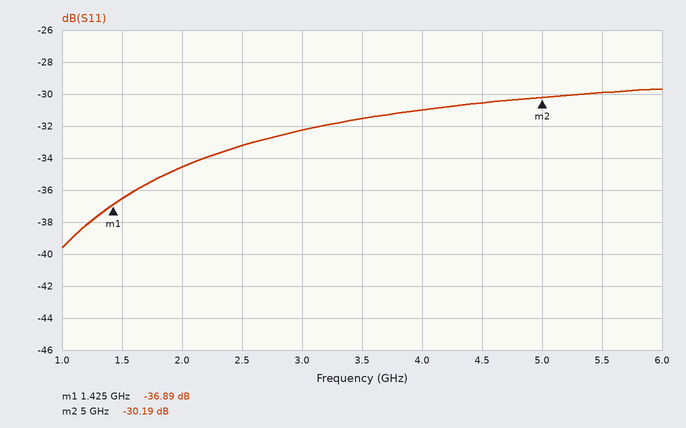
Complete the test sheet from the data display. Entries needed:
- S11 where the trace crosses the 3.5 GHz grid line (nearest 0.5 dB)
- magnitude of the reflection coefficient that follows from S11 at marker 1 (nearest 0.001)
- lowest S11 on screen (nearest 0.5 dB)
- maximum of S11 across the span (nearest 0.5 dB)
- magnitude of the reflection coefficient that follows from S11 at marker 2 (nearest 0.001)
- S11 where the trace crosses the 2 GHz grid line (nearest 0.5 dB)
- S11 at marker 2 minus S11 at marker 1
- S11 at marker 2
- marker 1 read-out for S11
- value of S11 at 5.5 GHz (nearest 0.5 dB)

-31.5 dB
0.014
-39.5 dB
-29.5 dB
0.031
-34.5 dB
6.70 dB
-30.19 dB
-36.89 dB
-30.0 dB
